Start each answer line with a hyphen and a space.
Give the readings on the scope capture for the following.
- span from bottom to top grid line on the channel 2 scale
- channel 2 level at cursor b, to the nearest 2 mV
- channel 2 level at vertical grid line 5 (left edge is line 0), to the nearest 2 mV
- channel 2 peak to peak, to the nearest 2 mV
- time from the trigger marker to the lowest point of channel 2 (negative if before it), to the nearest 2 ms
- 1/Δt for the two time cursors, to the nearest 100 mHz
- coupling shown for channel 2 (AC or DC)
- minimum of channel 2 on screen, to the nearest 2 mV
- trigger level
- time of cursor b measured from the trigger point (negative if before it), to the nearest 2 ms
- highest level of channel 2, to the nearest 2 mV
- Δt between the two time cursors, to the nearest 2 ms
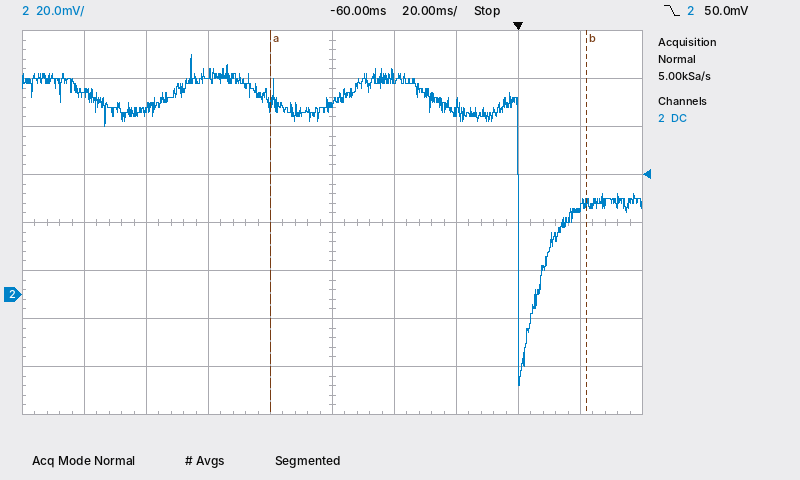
- 160 mV
- 38 mV
- 80 mV
- 138 mV
- 0 ms
- 9.8 Hz
- DC
- -38 mV
- 50.0 mV
- +22 ms
- 100 mV
- 102 ms
